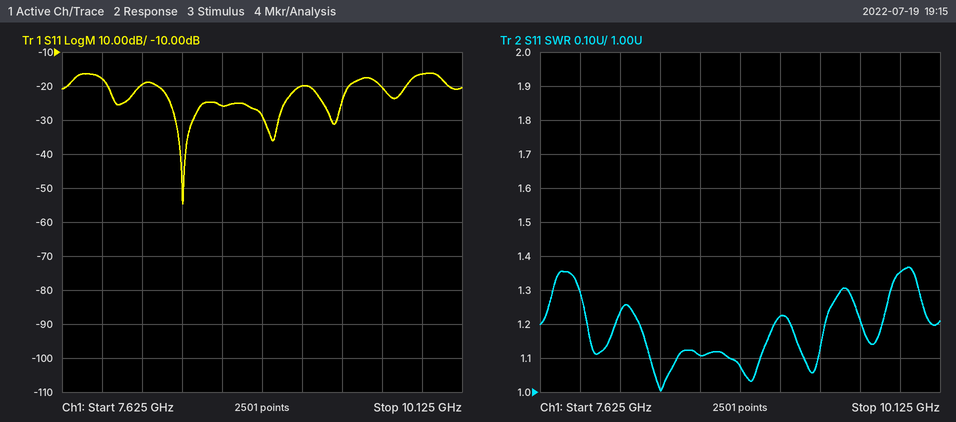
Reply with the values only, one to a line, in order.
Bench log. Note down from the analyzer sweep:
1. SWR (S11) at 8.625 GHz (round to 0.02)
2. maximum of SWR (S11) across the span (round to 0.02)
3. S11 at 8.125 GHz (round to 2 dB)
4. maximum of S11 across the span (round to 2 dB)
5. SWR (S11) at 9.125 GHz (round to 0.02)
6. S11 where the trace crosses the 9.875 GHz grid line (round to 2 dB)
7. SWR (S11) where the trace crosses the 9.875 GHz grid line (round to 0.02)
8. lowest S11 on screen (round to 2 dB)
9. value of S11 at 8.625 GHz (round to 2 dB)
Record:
1.10
1.36
-20 dB
-16 dB
1.22
-16 dB
1.36
-54 dB
-26 dB
